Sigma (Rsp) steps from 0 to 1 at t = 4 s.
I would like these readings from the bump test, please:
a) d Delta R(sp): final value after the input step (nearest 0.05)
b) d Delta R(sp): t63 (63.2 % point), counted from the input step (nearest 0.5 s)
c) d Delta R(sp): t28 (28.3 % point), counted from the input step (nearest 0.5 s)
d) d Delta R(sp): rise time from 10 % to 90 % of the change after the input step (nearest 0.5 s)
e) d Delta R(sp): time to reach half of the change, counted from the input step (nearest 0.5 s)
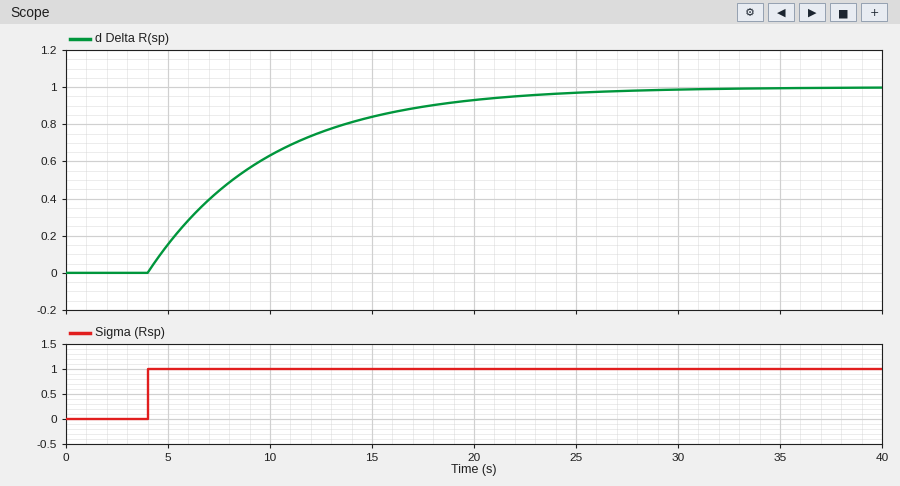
1.00
6.0 s
2.0 s
13.0 s
4.0 s
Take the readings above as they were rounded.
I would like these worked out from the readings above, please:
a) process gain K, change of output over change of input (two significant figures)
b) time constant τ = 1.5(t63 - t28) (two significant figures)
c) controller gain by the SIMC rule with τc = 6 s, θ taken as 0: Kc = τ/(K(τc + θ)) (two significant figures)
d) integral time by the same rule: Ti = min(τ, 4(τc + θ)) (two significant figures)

1.0
6.0 s
1.0
6.0 s
